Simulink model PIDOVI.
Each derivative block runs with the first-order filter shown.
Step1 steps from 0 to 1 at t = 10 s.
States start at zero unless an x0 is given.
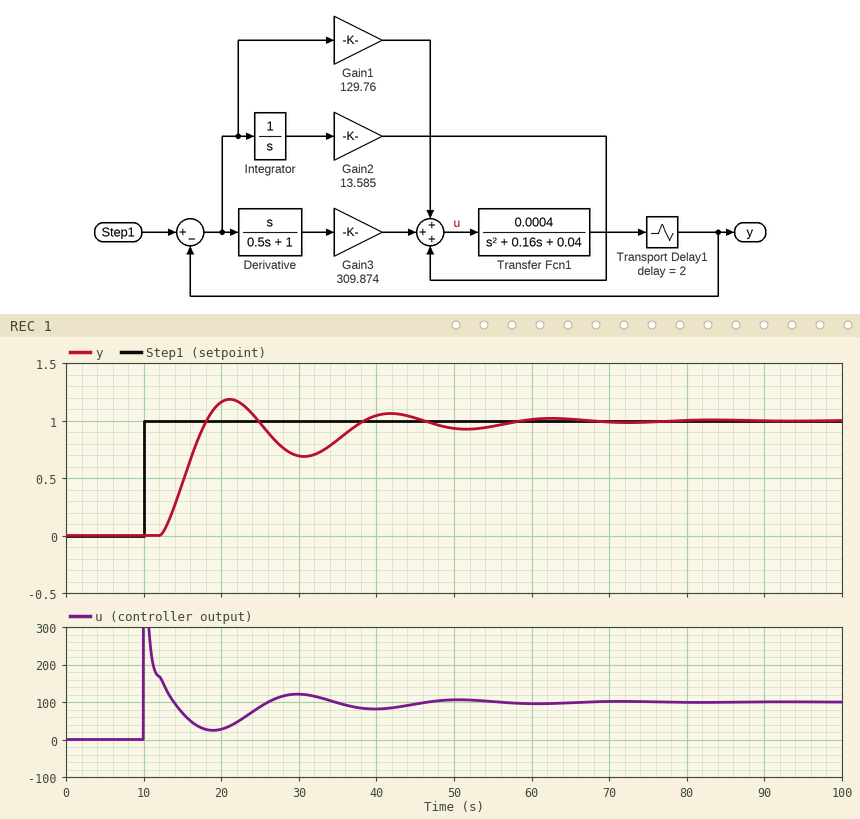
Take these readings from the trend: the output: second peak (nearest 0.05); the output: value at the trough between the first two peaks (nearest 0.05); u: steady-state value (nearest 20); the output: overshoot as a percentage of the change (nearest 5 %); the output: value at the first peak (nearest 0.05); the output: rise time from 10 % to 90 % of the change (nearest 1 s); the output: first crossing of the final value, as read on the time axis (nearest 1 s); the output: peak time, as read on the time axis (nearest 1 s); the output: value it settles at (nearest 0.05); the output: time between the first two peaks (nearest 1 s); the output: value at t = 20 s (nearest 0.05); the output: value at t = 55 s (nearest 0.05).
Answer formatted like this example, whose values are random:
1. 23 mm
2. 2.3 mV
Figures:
1. 1.05
2. 0.70
3. 100
4. 20 %
5. 1.20
6. 4 s
7. 18 s
8. 21 s
9. 1.00
10. 21 s
11. 1.15
12. 0.95
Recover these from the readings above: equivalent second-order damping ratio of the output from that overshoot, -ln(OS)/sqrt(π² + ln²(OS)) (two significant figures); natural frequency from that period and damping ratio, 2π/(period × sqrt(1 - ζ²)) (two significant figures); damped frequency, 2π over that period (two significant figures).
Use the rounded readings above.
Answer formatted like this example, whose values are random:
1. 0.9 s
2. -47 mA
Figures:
1. 0.46
2. 0.34 rad/s
3. 0.30 rad/s
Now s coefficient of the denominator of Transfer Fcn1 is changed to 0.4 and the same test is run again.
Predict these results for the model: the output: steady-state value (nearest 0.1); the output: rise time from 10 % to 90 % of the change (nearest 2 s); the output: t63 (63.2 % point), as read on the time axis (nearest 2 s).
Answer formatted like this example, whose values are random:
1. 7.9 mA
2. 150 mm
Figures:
1. 1.0
2. 10 s
3. 18 s
